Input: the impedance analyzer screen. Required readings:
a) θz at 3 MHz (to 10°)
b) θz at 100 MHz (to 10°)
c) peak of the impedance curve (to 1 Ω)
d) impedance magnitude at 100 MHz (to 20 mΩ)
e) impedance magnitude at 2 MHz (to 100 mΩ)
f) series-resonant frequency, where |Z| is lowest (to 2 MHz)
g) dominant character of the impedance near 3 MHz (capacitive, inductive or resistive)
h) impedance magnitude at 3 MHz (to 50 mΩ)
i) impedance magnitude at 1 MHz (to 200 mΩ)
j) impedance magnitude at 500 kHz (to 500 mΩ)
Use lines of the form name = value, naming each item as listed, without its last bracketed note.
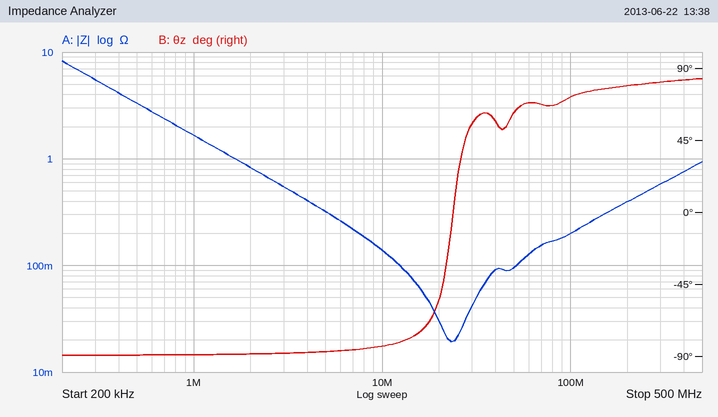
θz at 3 MHz = -90°
θz at 100 MHz = 70°
peak of the impedance curve = 8 Ω
impedance magnitude at 100 MHz = 200 mΩ
impedance magnitude at 2 MHz = 800 mΩ
series-resonant frequency, where |Z| is lowest = 24 MHz
dominant character of the impedance near 3 MHz = capacitive
impedance magnitude at 3 MHz = 550 mΩ
impedance magnitude at 1 MHz = 1.6 Ω
impedance magnitude at 500 kHz = 3.5 Ω
